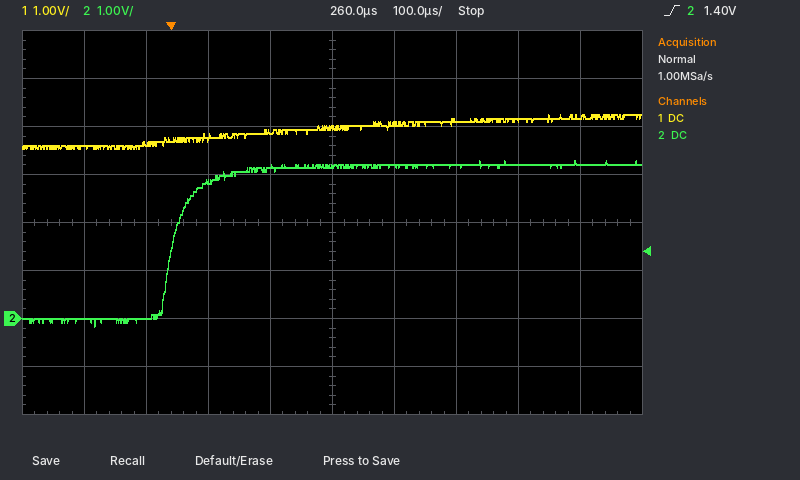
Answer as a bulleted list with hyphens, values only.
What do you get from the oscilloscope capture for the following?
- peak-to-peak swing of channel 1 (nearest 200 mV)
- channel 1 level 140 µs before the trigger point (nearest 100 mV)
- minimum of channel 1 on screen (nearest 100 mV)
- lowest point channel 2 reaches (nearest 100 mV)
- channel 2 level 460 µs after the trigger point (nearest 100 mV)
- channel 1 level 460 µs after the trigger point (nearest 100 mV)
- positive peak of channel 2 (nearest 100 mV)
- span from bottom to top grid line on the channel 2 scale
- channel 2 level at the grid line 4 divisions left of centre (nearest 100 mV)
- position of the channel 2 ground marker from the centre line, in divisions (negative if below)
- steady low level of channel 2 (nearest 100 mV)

- 800 mV
- 3.6 V
- 3.5 V
- -200 mV
- 3.2 V
- 4.1 V
- 3.3 V
- 8 V
- 0.0 V
- -2.0 div
- 0.0 V
